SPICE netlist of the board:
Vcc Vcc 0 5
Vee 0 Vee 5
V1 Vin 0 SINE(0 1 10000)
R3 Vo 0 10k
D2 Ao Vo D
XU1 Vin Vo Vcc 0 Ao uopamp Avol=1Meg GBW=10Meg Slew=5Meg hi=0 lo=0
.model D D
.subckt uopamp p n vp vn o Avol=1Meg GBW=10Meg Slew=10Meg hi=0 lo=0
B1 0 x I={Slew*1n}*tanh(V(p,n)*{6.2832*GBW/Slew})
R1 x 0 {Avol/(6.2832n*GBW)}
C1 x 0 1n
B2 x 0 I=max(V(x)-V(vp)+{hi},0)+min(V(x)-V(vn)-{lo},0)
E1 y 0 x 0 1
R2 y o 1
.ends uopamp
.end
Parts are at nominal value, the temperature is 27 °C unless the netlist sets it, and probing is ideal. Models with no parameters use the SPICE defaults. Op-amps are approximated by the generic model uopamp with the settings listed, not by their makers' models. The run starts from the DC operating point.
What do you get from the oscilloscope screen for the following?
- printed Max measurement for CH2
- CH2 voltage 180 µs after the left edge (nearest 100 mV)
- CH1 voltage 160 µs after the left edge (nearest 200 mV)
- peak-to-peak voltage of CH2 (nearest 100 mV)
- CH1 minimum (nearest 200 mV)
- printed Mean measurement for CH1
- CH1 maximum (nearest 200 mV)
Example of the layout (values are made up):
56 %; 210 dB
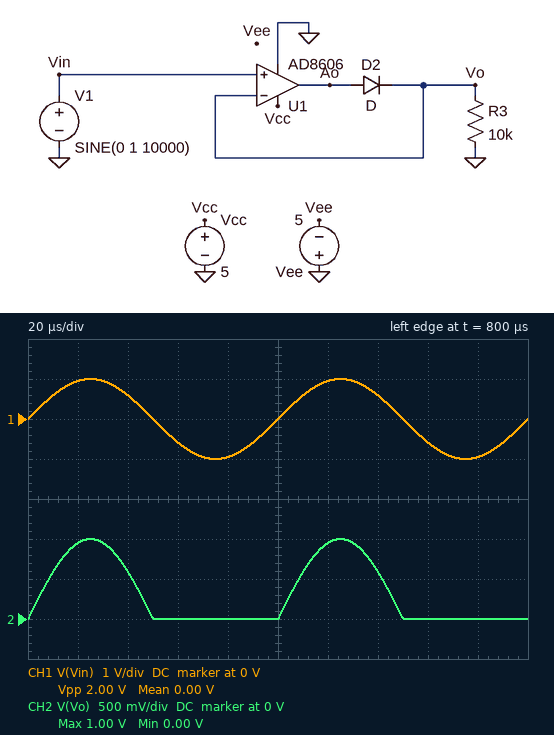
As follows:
1.00 V; 0 V; -600 mV; 1.0 V; -1.0 V; 0.00 V; 1.0 V
